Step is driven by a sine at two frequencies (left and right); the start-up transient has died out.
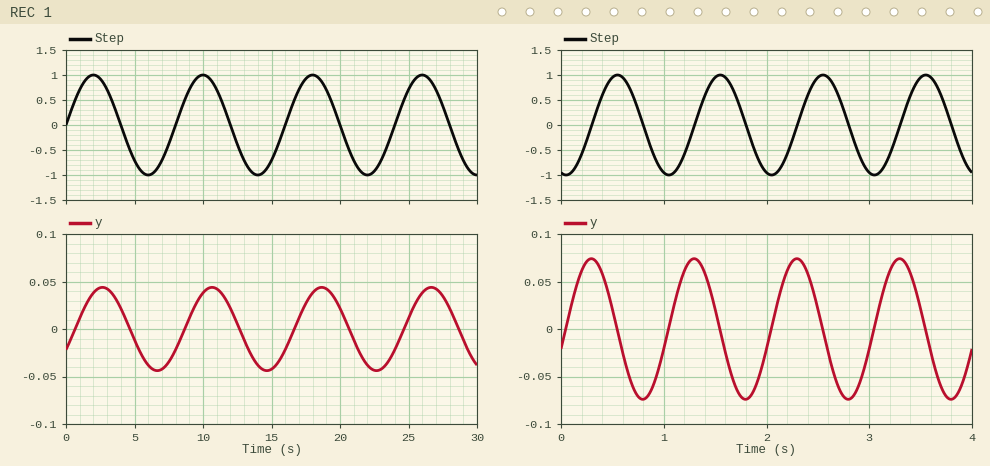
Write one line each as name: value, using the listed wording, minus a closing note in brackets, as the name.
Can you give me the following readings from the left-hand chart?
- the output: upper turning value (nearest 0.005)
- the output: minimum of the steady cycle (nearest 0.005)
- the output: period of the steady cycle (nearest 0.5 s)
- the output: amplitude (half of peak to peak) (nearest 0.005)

the output: upper turning value: 0.045
the output: minimum of the steady cycle: -0.045
the output: period of the steady cycle: 8.0 s
the output: amplitude (half of peak to peak): 0.045
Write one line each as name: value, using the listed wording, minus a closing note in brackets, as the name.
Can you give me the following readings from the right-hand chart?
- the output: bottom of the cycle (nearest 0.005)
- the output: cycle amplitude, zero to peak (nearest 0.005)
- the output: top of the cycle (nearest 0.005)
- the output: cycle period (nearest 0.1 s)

the output: bottom of the cycle: -0.075
the output: cycle amplitude, zero to peak: 0.075
the output: top of the cycle: 0.075
the output: cycle period: 1.0 s
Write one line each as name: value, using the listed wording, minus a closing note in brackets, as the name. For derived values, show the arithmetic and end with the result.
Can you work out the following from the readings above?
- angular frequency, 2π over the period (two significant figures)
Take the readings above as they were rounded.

angular frequency, 2π over the period: 2π / 1 = 6.3 rad/s
